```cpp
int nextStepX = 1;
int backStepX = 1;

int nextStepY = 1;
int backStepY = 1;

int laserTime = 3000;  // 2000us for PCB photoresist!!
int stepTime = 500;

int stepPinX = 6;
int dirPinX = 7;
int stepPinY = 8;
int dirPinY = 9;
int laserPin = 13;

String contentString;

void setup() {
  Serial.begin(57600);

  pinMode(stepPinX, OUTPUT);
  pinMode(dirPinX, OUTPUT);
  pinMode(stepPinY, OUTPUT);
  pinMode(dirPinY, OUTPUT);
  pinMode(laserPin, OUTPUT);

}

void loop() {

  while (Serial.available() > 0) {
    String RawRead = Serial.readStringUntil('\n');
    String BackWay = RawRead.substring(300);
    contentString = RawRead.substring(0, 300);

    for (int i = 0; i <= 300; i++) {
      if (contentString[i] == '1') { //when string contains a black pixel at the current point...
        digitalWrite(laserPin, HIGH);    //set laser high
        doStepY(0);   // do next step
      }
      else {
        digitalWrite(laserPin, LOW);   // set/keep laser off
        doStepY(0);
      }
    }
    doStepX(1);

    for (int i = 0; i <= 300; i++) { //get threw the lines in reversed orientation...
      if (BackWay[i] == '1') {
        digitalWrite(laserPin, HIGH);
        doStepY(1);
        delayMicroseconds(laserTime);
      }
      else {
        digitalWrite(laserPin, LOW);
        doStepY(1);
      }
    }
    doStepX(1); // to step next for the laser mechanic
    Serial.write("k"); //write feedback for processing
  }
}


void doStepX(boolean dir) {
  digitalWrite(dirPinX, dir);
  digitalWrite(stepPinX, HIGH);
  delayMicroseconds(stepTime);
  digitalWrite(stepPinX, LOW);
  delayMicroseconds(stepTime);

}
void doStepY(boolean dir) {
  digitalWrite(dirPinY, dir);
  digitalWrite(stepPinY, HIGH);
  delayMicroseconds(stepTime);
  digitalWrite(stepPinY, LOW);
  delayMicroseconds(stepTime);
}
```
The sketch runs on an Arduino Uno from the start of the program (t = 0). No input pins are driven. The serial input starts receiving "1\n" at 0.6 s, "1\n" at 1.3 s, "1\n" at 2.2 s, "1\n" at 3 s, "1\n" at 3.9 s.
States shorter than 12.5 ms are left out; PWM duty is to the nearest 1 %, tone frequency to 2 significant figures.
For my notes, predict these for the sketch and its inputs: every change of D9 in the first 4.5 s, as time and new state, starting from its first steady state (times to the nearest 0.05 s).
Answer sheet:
0 s low; 0.9 s high; 1.3 s low; 1.6 s high; 2.2 s low; 2.5 s high; 3 s low; 3.3 s high; 3.9 s low; 4.2 s high
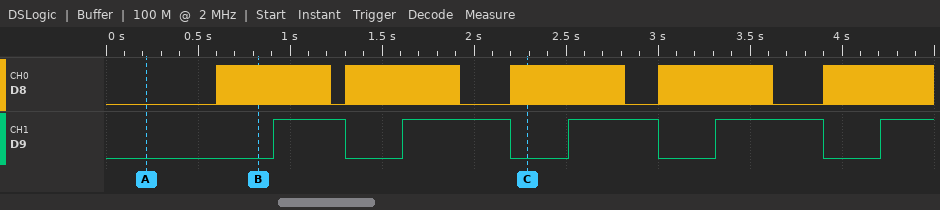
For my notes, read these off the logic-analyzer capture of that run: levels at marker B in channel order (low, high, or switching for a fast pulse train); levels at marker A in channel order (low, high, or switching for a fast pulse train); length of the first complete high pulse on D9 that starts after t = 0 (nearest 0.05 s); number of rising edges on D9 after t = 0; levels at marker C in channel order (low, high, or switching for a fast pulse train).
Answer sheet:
D8 switching, D9 low
D8 low, D9 low
0.40 s
5
D8 switching, D9 low
